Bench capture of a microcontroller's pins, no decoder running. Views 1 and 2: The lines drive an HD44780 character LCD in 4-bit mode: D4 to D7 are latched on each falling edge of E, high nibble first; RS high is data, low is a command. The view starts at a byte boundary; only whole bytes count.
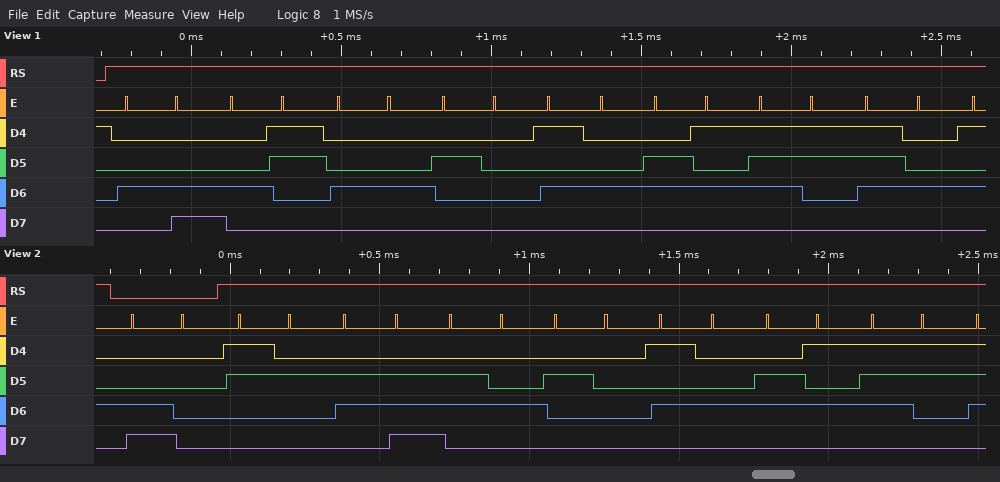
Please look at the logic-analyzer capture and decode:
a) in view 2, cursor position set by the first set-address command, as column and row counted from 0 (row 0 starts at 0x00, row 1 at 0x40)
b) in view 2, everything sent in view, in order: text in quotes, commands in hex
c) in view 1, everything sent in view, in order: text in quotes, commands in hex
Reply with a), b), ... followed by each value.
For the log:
a) column 0, row 1
b) 0xC0 "2nd Tes"
c) "LCD Test"
